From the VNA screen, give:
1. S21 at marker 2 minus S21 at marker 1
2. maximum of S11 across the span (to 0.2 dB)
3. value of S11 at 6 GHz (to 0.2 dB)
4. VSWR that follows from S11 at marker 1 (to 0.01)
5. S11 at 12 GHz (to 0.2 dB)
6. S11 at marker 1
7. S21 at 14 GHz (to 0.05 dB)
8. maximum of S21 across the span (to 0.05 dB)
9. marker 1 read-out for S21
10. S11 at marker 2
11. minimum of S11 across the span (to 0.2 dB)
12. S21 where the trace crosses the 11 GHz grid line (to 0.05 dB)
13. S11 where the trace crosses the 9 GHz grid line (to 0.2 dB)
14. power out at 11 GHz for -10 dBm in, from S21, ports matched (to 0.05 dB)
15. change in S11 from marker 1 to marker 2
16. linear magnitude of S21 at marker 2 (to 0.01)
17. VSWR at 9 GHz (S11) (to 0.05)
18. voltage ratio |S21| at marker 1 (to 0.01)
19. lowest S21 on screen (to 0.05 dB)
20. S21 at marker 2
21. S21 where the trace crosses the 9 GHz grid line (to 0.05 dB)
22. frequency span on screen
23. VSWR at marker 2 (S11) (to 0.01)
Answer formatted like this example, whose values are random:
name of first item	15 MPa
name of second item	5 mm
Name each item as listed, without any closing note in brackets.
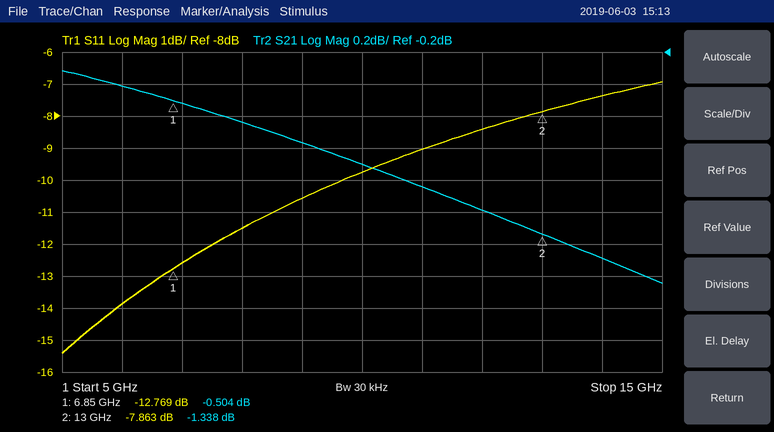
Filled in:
S21 at marker 2 minus S21 at marker 1	-0.834 dB
maximum of S11 across the span	-7.0 dB
value of S11 at 6 GHz	-13.8 dB
VSWR that follows from S11 at marker 1	1.60
S11 at 12 GHz	-8.4 dB
S11 at marker 1	-12.769 dB
S21 at 14 GHz	-1.50 dB
maximum of S21 across the span	-0.30 dB
marker 1 read-out for S21	-0.504 dB
S11 at marker 2	-7.863 dB
minimum of S11 across the span	-15.4 dB
S21 where the trace crosses the 11 GHz grid line	-1.05 dB
S11 where the trace crosses the 9 GHz grid line	-10.6 dB
power out at 11 GHz for -10 dBm in, from S21, ports matched	-11.05 dBm
change in S11 from marker 1 to marker 2	4.906 dB
linear magnitude of S21 at marker 2	0.86
VSWR at 9 GHz (S11)	1.85
voltage ratio |S21| at marker 1	0.94
lowest S21 on screen	-1.65 dB
S21 at marker 2	-1.338 dB
S21 where the trace crosses the 9 GHz grid line	-0.75 dB
frequency span on screen	10 GHz
VSWR at marker 2 (S11)	2.36
